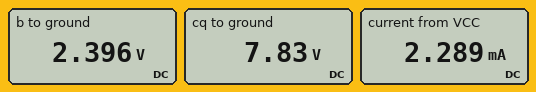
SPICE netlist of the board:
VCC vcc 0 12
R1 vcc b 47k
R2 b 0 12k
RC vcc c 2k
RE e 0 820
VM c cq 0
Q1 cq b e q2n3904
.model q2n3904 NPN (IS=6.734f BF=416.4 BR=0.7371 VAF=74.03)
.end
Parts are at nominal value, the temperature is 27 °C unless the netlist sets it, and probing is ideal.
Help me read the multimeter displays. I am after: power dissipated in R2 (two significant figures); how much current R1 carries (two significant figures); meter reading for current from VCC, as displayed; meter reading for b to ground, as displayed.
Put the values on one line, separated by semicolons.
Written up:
480 µW; 200 µA; 2.289 mA; 2.396 V
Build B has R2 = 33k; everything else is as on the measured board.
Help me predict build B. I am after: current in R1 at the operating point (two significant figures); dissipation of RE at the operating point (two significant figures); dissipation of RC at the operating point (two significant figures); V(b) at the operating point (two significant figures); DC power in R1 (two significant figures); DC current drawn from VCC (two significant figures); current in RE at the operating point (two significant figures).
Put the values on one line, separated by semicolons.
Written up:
170 µA; 15 mW; 35 mW; 4.2 V; 1.3 mW; 4.4 mA; 4.2 mA
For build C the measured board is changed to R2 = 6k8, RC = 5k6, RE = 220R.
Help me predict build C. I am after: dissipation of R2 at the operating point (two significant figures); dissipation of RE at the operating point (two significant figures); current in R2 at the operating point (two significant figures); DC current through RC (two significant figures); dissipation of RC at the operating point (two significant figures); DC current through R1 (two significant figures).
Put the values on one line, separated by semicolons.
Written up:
190 µW; 970 µW; 170 µA; 2.0 mA; 23 mW; 230 µA
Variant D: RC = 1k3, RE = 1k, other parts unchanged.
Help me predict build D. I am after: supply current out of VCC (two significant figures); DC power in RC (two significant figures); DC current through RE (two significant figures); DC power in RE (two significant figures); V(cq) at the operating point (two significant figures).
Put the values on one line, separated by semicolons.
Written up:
1.9 mA; 3.9 mW; 1.7 mA; 3.0 mW; 9.8 V
